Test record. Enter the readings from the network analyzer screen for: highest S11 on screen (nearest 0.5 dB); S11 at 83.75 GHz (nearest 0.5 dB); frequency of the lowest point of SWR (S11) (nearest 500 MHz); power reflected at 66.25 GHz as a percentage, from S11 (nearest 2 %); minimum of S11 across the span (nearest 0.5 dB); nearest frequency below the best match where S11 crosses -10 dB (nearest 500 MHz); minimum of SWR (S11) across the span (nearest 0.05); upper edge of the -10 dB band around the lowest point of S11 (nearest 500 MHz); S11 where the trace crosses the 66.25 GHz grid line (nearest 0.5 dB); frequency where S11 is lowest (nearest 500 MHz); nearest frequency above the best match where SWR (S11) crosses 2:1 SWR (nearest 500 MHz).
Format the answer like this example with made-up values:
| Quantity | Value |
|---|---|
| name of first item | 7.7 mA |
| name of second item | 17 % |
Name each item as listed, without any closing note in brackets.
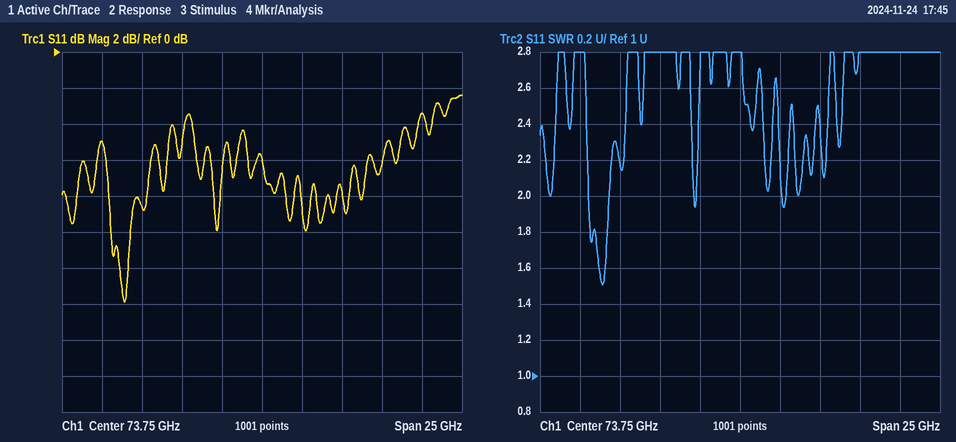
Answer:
| Quantity | Value |
|---|---|
| highest S11 on screen | -2.5 dB |
| S11 at 83.75 GHz | -3.5 dB |
| frequency of the lowest point of SWR (S11) | 65.0 GHz |
| power reflected at 66.25 GHz as a percentage, from S11 | 14 % |
| minimum of S11 across the span | -14.0 dB |
| nearest frequency below the best match where S11 crosses -10 dB | 64.5 GHz |
| minimum of SWR (S11) across the span | 1.50 |
| upper edge of the -10 dB band around the lowest point of S11 | 65.5 GHz |
| S11 where the trace crosses the 66.25 GHz grid line | -8.5 dB |
| frequency where S11 is lowest | 65.0 GHz |
| nearest frequency above the best match where SWR (S11) crosses 2:1 SWR | 65.5 GHz |
